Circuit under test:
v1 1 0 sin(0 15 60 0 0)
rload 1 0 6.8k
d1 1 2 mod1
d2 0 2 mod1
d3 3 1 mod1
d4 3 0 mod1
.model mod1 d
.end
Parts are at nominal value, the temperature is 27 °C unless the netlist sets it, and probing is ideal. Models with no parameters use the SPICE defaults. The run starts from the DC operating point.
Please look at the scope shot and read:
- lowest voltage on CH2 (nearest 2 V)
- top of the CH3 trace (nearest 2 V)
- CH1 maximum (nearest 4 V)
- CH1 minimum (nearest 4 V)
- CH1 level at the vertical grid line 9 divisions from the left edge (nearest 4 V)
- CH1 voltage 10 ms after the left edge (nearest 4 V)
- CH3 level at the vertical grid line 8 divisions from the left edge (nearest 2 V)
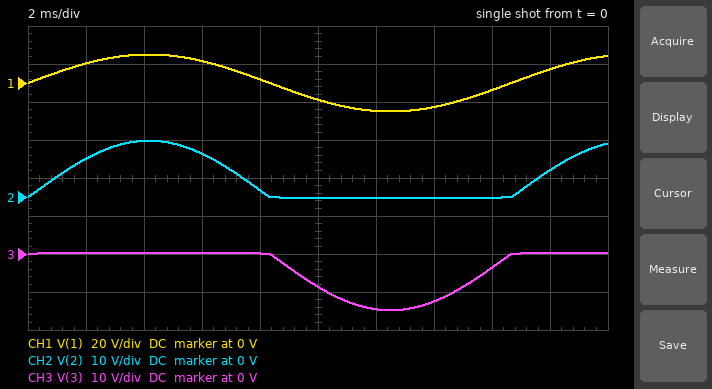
0 V
0 V
16 V
-16 V
8 V
-8 V
-4 V
